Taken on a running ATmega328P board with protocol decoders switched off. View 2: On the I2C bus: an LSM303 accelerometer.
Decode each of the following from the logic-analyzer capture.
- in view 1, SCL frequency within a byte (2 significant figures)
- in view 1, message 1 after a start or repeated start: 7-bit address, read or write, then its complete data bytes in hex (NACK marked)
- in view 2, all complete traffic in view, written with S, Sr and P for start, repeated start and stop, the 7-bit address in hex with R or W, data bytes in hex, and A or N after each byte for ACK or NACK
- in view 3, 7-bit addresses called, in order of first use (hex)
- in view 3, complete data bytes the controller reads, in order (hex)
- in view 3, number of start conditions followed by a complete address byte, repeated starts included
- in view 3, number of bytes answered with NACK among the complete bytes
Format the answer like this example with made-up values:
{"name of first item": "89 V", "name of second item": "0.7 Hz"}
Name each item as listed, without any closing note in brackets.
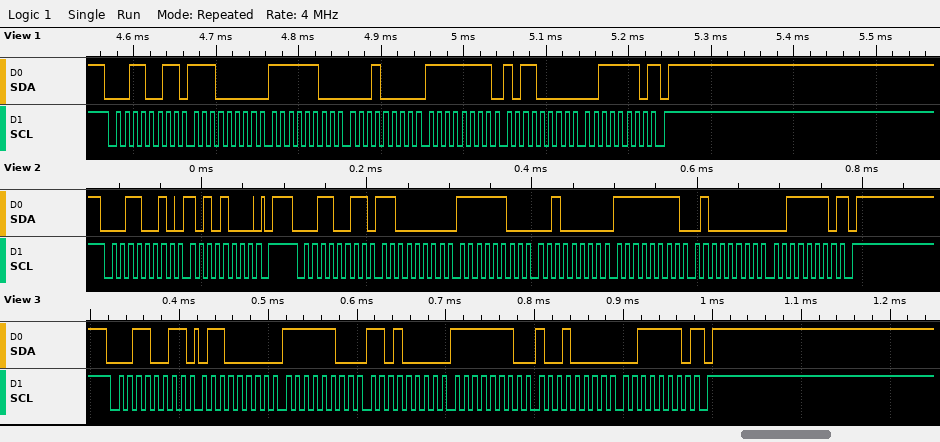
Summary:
{"in view 1, SCL frequency within a byte": "100 kHz", "in view 1, message 1 after a start or repeated start: 7-bit address, read or write, then its complete data bytes in hex": "0x19 read: E0 FC 10 FF B0 3E NACK", "in view 2, all complete traffic in view, written with S, Sr and P for start, repeated start and stop, the 7-bit address in hex with R or W, data bytes in hex, and A or N after each byte for ACK or NACK": "S 19W A A8 A P S 19R A C0 A FC A 20 A FF A 40 A 3E N P", "in view 3, 7-bit addresses called, in order of first use": "0x19", "in view 3, complete data bytes the controller reads, in order": "60 FC D0 FE 90 3E", "in view 3, number of start conditions followed by a complete address byte, repeated starts included": "1", "in view 3, number of bytes answered with NACK among the complete bytes": "1"}
